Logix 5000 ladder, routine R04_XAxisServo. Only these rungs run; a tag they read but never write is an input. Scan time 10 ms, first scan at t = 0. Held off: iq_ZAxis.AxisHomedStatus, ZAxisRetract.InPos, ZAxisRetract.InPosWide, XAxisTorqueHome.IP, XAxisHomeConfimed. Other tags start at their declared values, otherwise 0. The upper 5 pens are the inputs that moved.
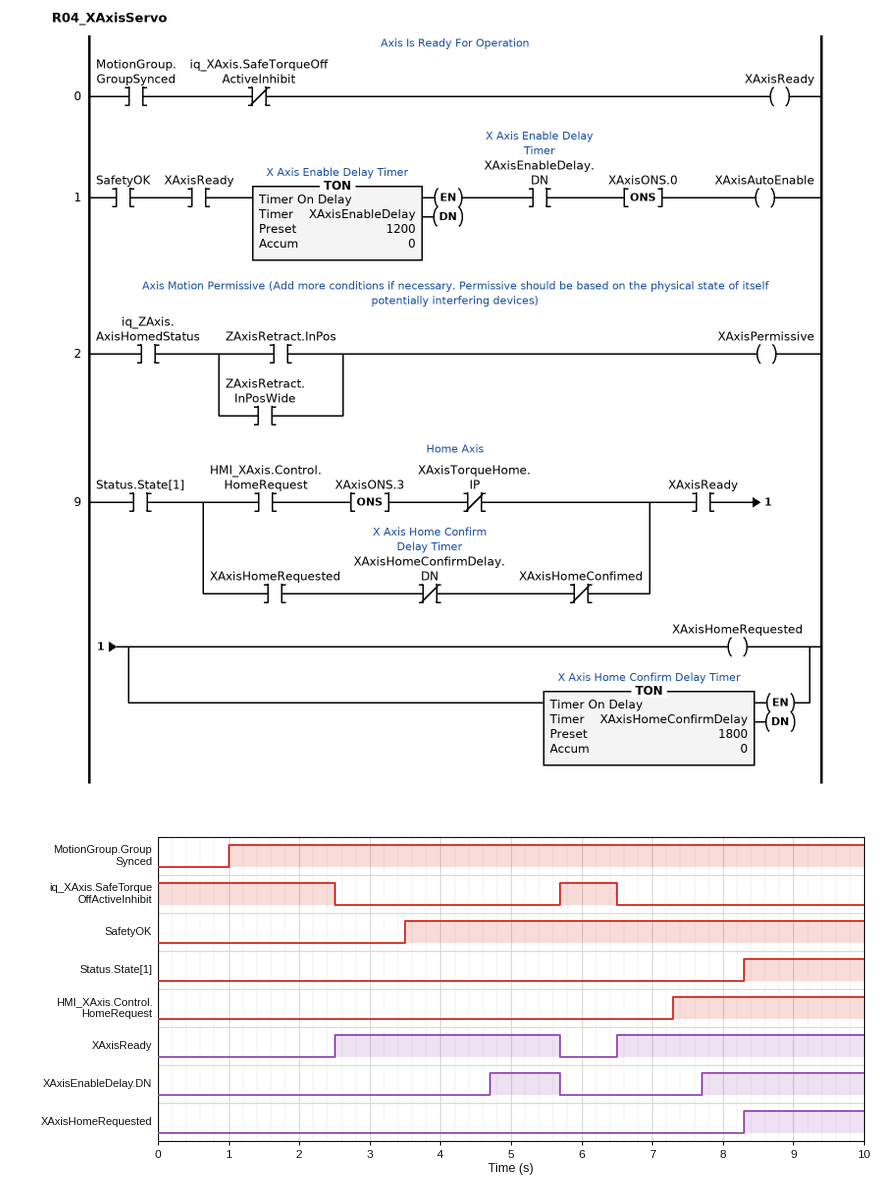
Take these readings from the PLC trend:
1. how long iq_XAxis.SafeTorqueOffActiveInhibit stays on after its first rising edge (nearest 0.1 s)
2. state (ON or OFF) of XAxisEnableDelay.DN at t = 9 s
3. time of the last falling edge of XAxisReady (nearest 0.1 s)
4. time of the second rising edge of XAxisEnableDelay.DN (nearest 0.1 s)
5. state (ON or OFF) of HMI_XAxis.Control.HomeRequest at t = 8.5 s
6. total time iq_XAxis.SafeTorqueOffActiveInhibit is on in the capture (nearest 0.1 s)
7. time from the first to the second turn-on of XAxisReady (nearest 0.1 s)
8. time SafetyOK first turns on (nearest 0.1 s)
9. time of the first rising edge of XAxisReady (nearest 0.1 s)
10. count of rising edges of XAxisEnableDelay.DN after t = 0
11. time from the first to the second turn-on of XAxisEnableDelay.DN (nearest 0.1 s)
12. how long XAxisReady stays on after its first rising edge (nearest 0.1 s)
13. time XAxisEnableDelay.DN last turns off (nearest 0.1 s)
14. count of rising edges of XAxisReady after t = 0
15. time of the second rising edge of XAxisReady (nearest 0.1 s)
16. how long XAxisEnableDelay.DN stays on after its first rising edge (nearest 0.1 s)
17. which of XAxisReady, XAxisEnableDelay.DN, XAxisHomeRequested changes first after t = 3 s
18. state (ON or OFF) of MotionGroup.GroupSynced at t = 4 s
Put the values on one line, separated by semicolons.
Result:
0.8 s; ON; 5.7 s; 7.7 s; ON; 3.3 s; 4.0 s; 3.5 s; 2.5 s; 2; 3.0 s; 3.2 s; 5.7 s; 2; 6.5 s; 1.0 s; XAxisEnableDelay.DN; ON
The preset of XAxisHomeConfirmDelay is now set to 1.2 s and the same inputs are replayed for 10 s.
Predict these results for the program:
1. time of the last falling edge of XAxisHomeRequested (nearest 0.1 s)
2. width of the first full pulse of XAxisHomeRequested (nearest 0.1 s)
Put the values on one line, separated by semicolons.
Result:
9.5 s; 1.2 s
